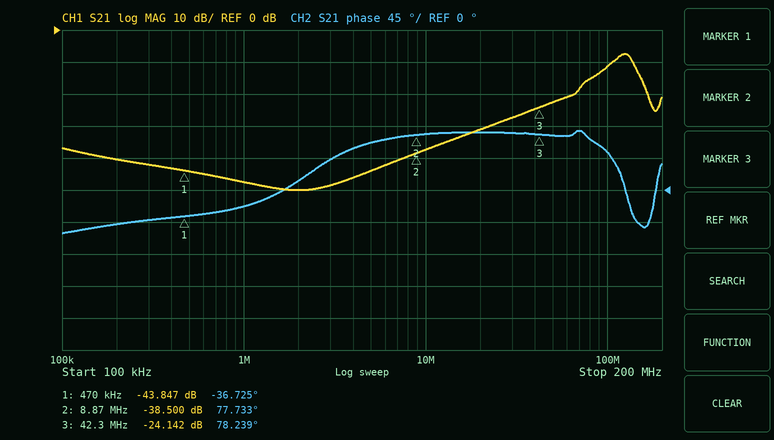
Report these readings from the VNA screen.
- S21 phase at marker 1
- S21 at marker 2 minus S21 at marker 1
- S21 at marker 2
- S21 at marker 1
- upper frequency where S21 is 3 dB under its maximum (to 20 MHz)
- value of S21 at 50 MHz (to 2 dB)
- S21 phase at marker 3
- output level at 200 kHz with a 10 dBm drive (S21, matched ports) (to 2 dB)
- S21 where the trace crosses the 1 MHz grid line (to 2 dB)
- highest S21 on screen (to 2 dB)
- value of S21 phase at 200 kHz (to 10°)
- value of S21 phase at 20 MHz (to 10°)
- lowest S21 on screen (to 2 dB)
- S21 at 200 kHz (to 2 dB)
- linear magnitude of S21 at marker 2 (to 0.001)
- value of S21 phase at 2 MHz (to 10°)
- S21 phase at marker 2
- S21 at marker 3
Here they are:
-36.725°
5.347 dB
-38.500 dB
-43.847 dB
140 MHz
-22 dB
78.239°
-30 dBm
-48 dB
-8 dB
-50°
80°
-50 dB
-40 dB
0.012
10°
77.733°
-24.142 dB
